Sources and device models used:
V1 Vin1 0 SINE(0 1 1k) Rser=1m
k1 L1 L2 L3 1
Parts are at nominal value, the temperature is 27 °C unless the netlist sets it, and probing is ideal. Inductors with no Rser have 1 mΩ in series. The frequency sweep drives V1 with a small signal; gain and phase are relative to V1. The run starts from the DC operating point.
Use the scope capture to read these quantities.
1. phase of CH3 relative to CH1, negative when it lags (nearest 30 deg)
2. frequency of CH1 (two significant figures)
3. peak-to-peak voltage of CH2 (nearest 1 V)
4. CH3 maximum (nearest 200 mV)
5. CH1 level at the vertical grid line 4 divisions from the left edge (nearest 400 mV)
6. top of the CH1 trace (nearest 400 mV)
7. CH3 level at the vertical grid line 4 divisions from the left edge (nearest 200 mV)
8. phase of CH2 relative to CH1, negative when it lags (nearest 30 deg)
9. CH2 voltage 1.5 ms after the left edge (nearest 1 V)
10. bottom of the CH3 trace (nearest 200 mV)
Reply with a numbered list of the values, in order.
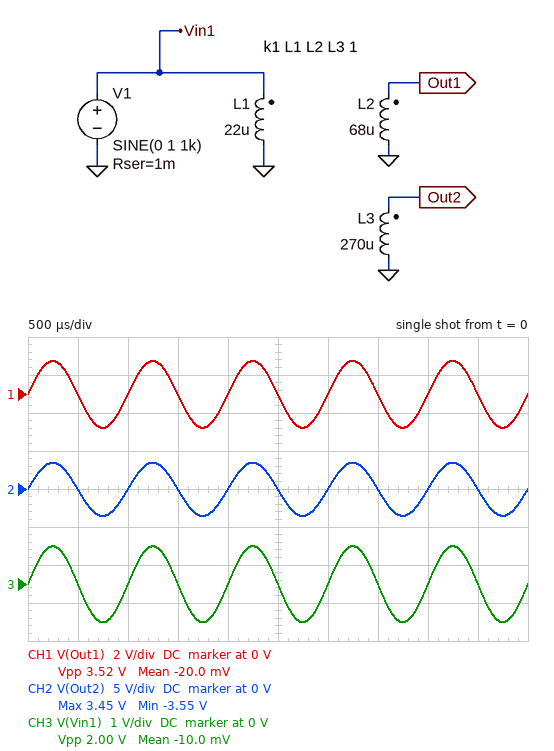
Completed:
1. 0 deg
2. 1.0 kHz
3. 7 V
4. 1.0 V
5. 0 V
6. 1.6 V
7. 0 V
8. 0 deg
9. 0 V
10. -1.0 V
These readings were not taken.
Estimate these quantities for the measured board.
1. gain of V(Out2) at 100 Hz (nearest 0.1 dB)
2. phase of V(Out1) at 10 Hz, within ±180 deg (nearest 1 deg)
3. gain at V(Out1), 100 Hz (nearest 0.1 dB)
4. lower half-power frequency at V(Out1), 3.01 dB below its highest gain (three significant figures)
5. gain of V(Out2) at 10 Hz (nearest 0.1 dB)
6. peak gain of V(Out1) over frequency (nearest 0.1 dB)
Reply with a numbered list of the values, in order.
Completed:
1. 10.8 dB
2. 55 deg
3. 4.8 dB
4. 14.5 Hz
5. 6.0 dB
6. 4.9 dB
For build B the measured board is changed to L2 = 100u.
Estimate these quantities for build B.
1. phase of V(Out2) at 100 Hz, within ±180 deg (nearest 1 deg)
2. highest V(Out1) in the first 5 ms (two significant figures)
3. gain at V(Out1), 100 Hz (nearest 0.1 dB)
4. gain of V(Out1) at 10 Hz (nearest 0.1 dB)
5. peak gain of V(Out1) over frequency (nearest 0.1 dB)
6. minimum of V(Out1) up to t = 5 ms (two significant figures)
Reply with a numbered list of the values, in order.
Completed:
1. 8 deg
2. 2.1 V
3. 6.5 dB
4. 1.7 dB
5. 6.6 dB
6. -2.2 V
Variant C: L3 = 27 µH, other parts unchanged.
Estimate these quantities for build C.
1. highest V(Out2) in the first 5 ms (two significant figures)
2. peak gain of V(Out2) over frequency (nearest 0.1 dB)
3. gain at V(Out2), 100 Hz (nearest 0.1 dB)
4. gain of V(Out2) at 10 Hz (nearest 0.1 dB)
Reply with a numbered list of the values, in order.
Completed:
1. 1.1 V
2. 0.9 dB
3. 0.8 dB
4. -4.0 dB
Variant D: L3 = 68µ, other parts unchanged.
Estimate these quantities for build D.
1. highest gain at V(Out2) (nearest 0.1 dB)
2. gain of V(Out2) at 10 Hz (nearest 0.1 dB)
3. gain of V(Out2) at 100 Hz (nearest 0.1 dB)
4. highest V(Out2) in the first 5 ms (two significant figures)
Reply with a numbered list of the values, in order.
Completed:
1. 4.9 dB
2. 0 dB
3. 4.8 dB
4. 1.7 V
